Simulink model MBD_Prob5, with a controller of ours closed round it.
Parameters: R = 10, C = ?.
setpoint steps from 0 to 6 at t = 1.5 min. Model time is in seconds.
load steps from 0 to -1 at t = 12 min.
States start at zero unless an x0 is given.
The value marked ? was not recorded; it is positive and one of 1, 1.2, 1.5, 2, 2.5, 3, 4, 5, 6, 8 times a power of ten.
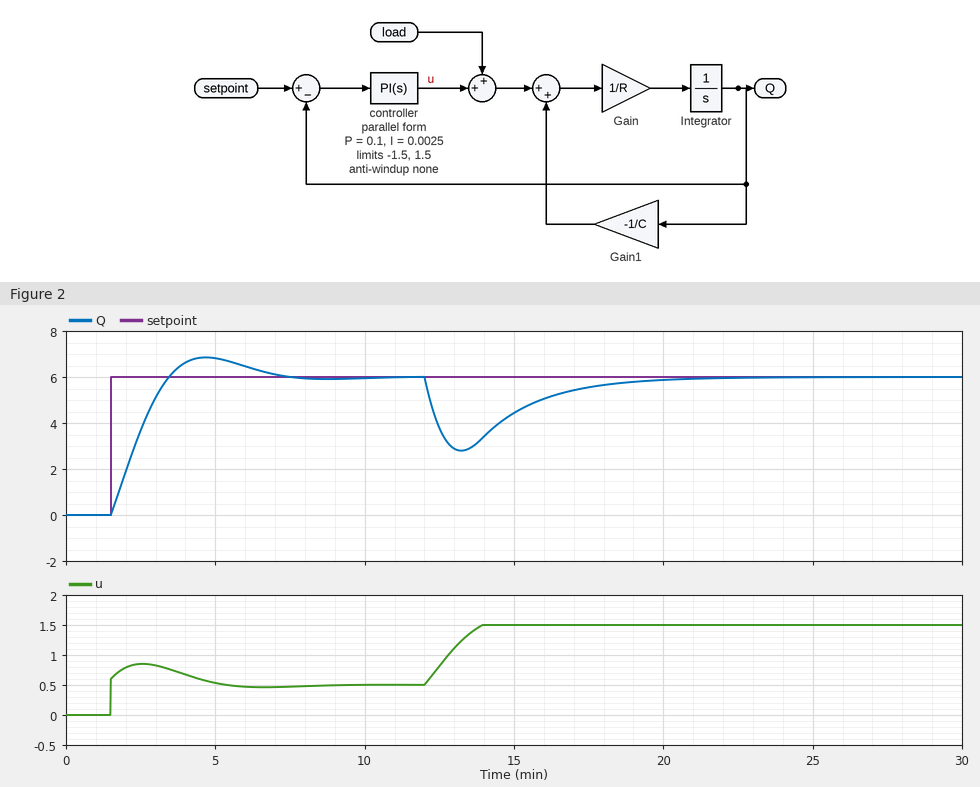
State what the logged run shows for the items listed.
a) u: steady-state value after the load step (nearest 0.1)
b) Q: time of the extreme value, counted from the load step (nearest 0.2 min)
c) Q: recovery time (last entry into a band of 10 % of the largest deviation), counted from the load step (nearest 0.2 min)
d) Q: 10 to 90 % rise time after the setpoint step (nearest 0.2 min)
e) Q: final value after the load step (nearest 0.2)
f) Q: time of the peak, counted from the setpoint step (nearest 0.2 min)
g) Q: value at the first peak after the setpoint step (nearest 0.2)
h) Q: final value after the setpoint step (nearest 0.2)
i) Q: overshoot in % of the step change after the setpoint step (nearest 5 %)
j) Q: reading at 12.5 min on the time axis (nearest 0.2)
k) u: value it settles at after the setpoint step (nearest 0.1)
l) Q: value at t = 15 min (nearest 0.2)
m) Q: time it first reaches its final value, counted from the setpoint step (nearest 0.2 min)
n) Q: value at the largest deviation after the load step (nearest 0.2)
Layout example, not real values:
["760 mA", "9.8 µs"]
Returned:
["1.5", "1.2 min", "6.2 min", "1.4 min", "6.0", "3.2 min", "6.8", "6.0", "15 %", "3.8", "0.5", "4.4", "2.0 min", "2.8"]
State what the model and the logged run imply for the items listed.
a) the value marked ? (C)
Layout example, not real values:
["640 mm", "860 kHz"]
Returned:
["12"]
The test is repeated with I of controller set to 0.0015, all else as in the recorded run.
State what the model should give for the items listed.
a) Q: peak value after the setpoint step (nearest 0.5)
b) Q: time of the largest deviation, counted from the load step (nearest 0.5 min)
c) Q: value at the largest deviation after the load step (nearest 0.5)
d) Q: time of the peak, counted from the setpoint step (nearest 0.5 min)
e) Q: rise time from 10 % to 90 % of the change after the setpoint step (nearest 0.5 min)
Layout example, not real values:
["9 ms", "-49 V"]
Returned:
["6.5", "1.5 min", "2.5", "4.5 min", "2.0 min"]
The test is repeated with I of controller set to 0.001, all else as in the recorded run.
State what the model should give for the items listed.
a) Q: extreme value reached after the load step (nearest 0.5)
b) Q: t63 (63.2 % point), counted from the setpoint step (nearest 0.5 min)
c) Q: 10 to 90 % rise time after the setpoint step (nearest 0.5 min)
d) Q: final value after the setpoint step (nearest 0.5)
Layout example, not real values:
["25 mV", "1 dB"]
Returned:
["2.0", "1.5 min", "3.0 min", "6.0"]
